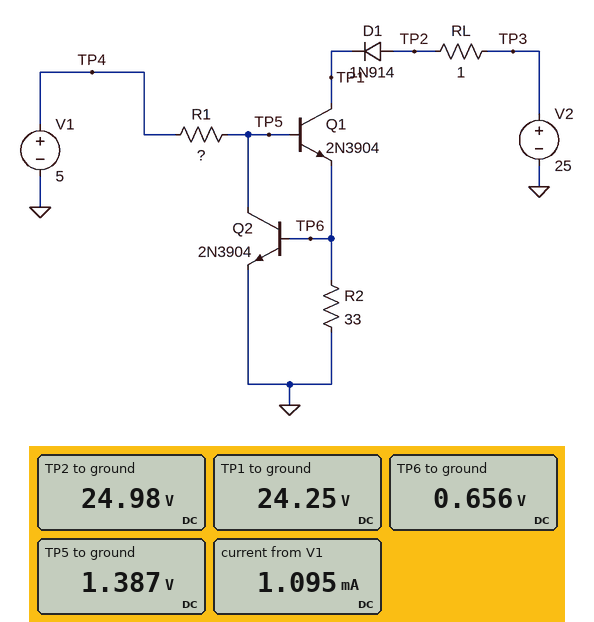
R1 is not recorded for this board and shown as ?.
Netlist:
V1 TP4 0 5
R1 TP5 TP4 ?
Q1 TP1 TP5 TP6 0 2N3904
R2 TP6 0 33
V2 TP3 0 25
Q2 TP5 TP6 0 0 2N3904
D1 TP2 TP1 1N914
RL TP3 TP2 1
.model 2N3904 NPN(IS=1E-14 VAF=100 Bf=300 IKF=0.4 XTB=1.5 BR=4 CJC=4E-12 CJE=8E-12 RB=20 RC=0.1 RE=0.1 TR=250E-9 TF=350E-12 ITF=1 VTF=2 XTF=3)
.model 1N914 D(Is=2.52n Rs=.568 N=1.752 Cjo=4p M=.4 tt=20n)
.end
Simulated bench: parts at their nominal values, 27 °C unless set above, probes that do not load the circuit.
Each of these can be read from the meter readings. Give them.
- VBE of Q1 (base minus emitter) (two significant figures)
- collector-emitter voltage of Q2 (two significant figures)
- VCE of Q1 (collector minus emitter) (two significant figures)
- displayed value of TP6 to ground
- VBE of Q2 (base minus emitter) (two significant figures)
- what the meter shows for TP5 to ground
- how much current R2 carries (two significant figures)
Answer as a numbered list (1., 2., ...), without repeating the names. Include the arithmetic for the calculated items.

1. 1.387 V - 656 mV = 730 mV
2. 1.387 V = 1.4 V
3. 24.25 V - 656 mV = 24 V
4. 0.656 V
5. 656 mV = 660 mV
6. 1.387 V
7. (656 mV) / 33 Ω = 20 mA
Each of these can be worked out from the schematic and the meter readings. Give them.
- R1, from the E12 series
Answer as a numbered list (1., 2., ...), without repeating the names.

1. 3.3 kΩ
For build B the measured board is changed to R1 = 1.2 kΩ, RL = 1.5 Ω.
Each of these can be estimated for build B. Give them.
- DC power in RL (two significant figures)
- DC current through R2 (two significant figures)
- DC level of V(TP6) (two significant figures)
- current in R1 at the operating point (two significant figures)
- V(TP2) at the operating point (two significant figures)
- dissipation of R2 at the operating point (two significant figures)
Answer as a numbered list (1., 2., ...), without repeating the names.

1. 640 µW
2. 21 mA
3. 680 mV
4. 3.0 mA
5. 25 V
6. 14 mW
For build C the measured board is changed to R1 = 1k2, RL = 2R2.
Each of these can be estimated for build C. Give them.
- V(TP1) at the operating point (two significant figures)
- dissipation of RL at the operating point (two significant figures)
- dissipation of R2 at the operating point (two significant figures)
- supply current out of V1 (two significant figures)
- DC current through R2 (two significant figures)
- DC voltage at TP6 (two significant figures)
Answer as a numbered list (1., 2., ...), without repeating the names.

1. 24 V
2. 940 µW
3. 14 mW
4. 3.0 mA
5. 21 mA
6. 680 mV
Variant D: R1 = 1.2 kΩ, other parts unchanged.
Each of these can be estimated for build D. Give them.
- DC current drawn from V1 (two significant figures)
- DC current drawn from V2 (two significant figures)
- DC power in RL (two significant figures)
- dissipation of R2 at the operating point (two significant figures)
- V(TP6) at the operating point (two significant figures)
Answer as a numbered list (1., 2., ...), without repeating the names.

1. 3.0 mA
2. 21 mA
3. 430 µW
4. 14 mW
5. 680 mV
